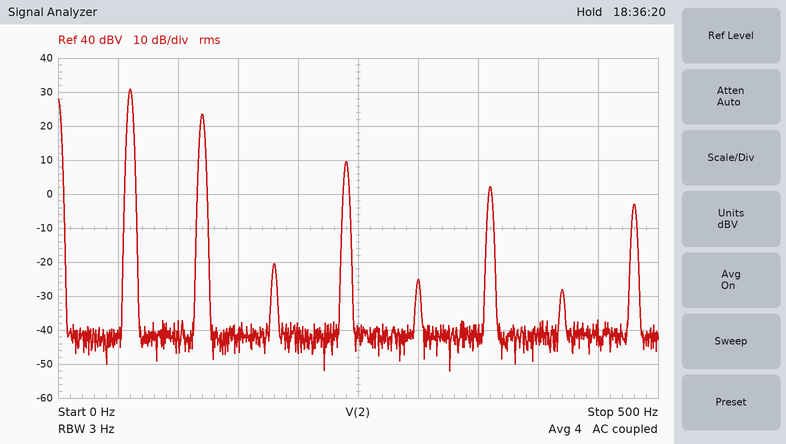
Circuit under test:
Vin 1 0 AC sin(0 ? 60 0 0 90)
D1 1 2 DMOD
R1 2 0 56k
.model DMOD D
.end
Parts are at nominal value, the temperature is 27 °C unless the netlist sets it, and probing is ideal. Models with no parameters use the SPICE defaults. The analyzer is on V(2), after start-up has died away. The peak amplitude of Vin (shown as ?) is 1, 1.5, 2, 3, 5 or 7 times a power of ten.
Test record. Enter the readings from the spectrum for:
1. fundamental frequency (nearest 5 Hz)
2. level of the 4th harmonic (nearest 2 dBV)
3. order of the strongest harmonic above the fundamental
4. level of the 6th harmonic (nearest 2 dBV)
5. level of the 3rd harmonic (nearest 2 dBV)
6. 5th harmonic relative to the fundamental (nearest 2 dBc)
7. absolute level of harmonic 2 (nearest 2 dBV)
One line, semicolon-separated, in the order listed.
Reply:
60 Hz; 10 dBV; 2; 2 dBV; -20 dBV; -56 dBc; 24 dBV
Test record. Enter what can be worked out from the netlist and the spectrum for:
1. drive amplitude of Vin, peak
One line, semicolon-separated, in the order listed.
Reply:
100 V
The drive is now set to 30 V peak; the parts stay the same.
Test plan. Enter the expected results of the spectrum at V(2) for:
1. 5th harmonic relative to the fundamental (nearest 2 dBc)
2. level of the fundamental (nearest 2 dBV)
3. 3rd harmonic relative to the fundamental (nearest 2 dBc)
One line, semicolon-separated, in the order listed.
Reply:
-46 dBc; 20 dBV; -42 dBc
